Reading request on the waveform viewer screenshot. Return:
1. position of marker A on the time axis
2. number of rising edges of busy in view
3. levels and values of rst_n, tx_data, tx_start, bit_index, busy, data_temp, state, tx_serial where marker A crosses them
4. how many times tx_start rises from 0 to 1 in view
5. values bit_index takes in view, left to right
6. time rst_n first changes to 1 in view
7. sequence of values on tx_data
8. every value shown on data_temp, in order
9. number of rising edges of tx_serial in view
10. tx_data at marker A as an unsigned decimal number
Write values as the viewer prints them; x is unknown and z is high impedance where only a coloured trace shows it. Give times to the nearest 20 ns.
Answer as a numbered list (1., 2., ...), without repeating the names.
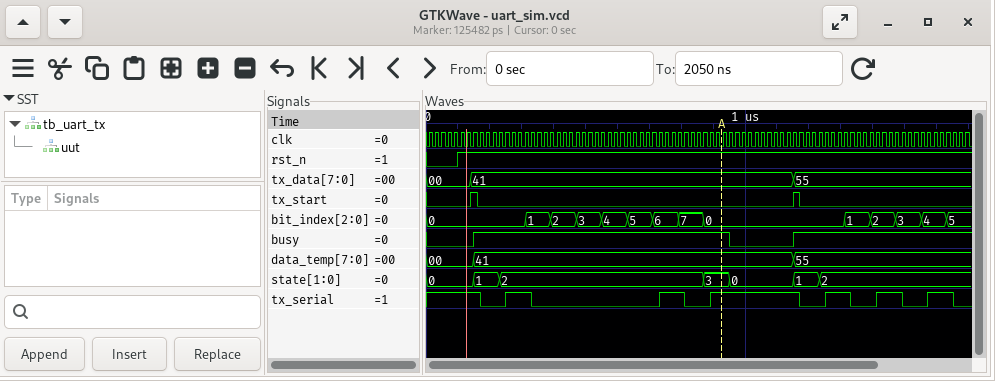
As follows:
1. 920 ns
2. 2
3. rst_n=1, tx_data=41, tx_start=0, bit_index=0, busy=1, data_temp=41, state=3, tx_serial=1
4. 2
5. 0, 1, 2, 3, 4, 5, 6, 7, 0, 1, 2, 3, 4, 5
6. 100 ns
7. 00, 41, 55
8. 00, 41, 55
9. 6
10. 65
